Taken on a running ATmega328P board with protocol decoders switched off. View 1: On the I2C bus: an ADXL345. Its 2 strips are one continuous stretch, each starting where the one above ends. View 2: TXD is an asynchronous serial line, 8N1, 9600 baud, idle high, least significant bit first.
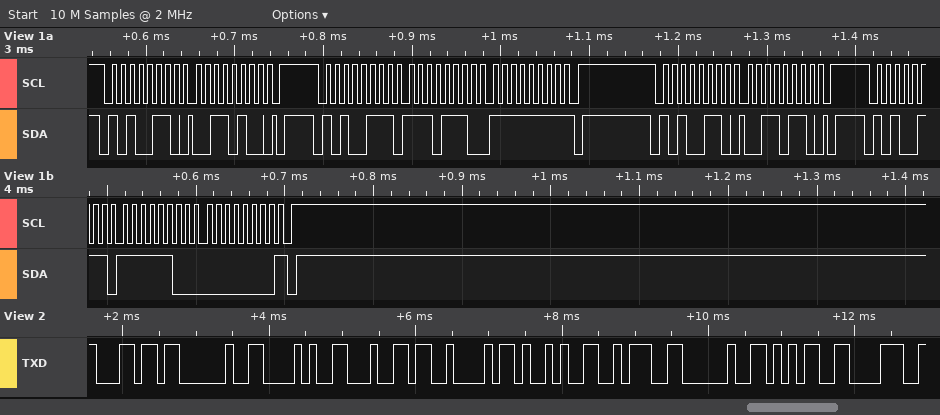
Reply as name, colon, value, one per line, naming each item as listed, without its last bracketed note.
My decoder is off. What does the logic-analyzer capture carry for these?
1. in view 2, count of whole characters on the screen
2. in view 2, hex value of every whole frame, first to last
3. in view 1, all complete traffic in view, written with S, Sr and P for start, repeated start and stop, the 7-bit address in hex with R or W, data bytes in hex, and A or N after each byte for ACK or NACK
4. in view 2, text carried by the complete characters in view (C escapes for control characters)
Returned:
in view 2, count of whole characters on the screen: 10
in view 2, hex value of every whole frame, first to last: 6C 20 28 64 42 29 3A 20 35 38
in view 1, all complete traffic in view, written with S, Sr and P for start, repeated start and stop, the 7-bit address in hex with R or W, data bytes in hex, and A or N after each byte for ACK or NACK: S 53W A 34 A P S 53R A EE A FF N P S 53W A 36 A P S 53R A FC A 00 N P
in view 2, text carried by the complete characters in view: "l (dB): 58"
